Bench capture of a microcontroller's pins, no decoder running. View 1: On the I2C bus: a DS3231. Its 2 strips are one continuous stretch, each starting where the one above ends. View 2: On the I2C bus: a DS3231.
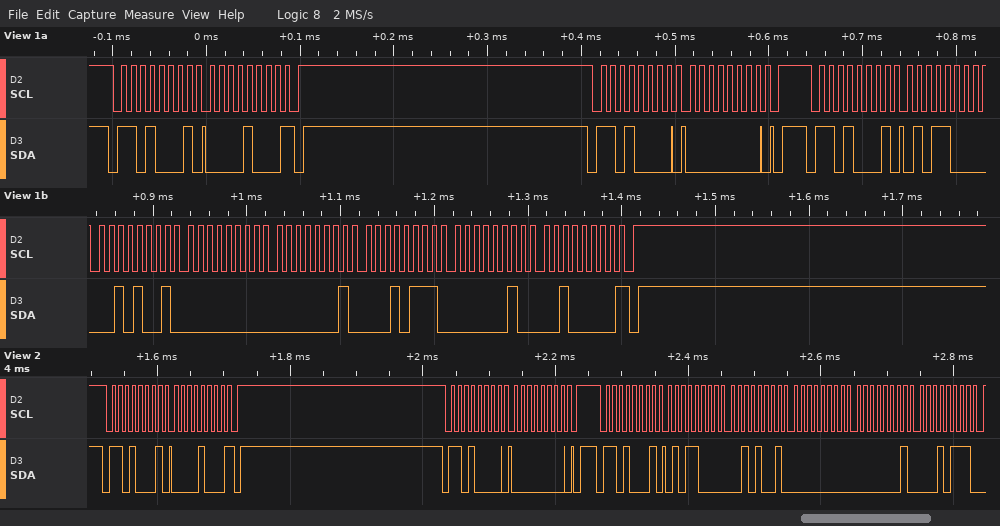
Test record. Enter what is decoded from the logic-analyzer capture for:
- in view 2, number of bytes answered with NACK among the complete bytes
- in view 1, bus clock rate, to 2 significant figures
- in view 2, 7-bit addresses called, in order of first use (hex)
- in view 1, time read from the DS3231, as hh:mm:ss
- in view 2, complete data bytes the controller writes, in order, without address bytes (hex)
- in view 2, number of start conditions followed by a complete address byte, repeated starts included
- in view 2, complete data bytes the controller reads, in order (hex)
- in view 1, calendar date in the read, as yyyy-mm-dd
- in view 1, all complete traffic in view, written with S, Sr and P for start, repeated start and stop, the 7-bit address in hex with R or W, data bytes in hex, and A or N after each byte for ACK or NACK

1
100 kHz
0x68
00:29:58
00
3
08 58 29 00 01 17
2020-02-17
S 68R A 08 N P S 68W A 00 A P S 68R A 58 A 29 A 00 A 01 A 17 A 02 A 20 N P
